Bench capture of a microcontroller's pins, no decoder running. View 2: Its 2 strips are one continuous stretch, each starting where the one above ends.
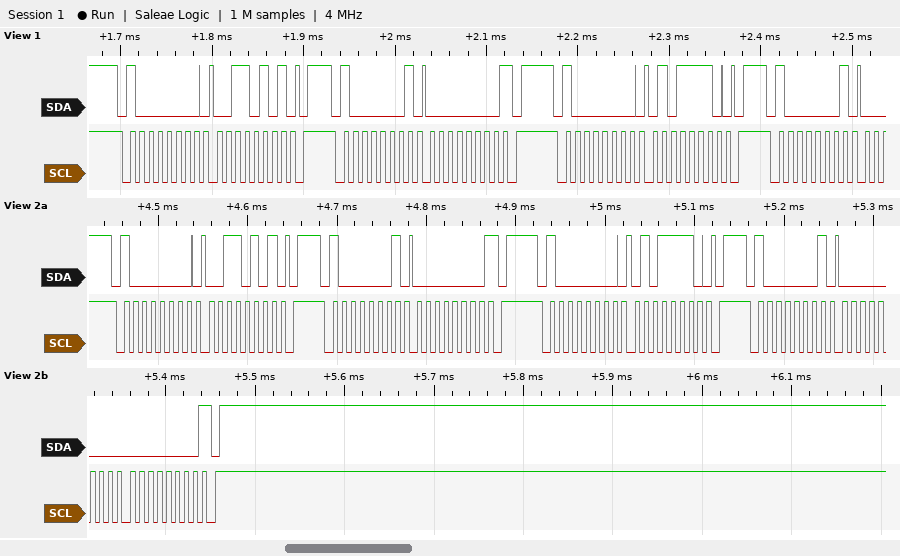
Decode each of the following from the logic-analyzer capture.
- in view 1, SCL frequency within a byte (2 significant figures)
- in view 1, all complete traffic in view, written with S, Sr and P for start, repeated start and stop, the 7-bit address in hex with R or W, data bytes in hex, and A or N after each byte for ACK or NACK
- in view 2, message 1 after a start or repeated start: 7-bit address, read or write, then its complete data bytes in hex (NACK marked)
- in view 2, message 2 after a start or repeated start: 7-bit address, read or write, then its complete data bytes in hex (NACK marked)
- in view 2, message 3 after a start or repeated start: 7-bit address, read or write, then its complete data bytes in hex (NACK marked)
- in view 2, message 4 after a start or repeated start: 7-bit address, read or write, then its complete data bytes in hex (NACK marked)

100 kHz
S 40W A 35 A P S 40R A 00 N P S 40W A 5E A P S 40R A
0x40 write: 35
0x40 read: 00 NACK
0x40 write: 5E
0x40 read: 00 00 NACK
